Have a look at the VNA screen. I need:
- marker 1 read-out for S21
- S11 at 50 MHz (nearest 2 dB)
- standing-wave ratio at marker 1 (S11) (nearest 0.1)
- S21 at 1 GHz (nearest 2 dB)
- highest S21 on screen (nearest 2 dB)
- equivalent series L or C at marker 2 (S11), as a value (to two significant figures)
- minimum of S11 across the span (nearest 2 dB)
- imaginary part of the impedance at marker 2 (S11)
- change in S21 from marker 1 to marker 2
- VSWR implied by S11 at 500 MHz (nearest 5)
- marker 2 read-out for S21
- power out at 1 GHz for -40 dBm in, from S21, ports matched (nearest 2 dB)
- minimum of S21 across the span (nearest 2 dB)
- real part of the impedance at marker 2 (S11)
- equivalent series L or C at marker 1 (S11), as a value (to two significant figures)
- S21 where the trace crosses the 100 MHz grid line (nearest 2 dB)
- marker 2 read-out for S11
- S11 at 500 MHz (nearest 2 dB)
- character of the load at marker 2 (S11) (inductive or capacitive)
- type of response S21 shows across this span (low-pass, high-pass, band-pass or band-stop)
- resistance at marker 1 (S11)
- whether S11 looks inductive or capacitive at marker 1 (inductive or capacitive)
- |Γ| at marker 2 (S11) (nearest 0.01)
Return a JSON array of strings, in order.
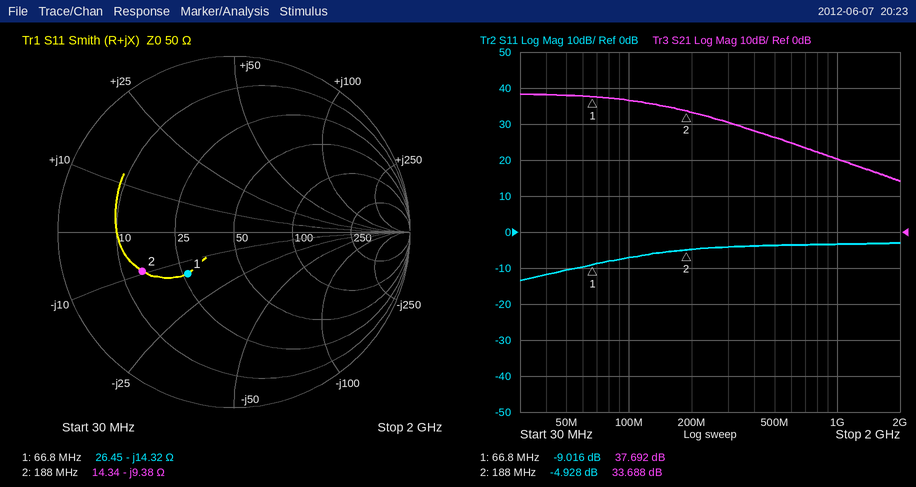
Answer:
["37.692 dB", "-10 dB", "2.1", "20 dB", "38 dB", "90 pF", "-14 dB", "-9.38 Ω", "-4.004 dB", "5", "33.688 dB", "-20 dBm", "14 dB", "14.34 Ω", "170 pF", "36 dB", "-4.928 dB", "-4 dB", "capacitive", "low-pass", "26.45 Ω", "capacitive", "0.57"]
